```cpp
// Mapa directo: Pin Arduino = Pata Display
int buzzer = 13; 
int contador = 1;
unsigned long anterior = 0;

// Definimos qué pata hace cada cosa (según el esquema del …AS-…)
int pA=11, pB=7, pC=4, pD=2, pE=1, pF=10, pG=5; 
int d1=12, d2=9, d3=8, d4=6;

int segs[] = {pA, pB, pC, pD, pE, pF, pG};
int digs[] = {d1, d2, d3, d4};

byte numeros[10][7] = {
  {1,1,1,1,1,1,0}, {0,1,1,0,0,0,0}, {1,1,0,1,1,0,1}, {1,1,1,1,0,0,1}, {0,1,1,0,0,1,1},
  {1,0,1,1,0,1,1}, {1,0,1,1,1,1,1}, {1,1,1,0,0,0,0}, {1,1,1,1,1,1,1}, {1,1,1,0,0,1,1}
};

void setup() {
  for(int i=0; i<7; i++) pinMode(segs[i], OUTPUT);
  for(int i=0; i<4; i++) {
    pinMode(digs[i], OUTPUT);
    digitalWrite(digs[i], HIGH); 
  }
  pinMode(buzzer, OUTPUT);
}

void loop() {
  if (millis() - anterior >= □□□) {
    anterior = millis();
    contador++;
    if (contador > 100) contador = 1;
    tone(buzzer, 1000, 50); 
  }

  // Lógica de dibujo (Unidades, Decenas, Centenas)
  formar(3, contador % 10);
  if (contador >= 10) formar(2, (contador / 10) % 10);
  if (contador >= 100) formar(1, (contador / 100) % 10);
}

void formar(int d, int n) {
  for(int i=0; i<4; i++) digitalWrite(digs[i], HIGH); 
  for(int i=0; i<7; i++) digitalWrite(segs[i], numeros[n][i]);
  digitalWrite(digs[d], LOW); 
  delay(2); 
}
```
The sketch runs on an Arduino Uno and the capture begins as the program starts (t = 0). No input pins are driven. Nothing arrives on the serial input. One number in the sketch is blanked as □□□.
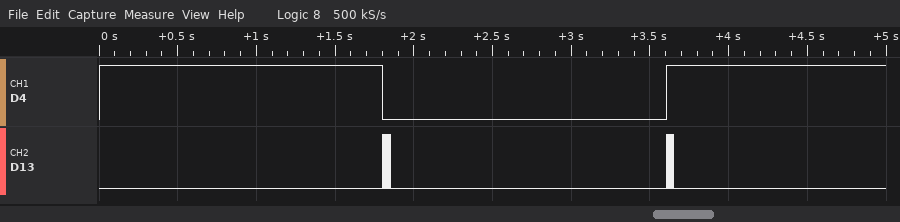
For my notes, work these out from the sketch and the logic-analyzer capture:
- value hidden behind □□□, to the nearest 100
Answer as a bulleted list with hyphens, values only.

- 1800
